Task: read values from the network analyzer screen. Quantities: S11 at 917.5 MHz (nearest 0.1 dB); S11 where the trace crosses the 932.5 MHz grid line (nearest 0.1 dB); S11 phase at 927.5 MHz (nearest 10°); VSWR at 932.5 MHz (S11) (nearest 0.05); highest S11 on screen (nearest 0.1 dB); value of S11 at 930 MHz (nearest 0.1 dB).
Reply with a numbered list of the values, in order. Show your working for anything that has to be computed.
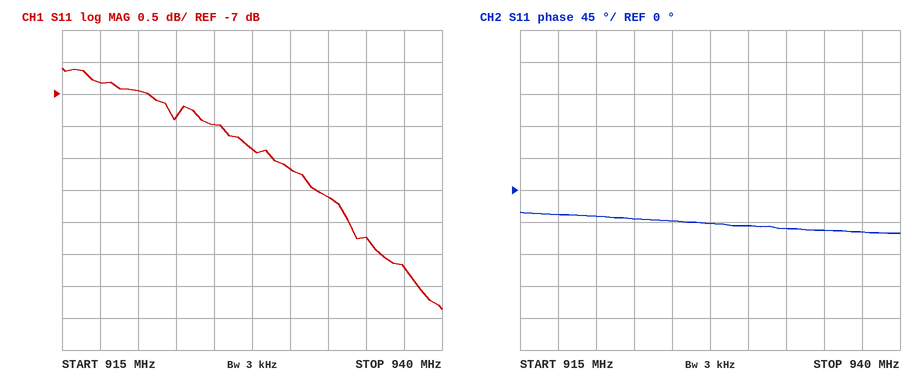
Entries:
1. -6.8 dB
2. -8.6 dB
3. -50°
4. |Γ| = 10^(-8.6/20) = 0.3715; VSWR = (1 + 0.3715)/(1 − 0.3715) ≈ 2.18, so 2.20 to the nearest 0.05
5. -6.6 dB
6. -8.2 dB
